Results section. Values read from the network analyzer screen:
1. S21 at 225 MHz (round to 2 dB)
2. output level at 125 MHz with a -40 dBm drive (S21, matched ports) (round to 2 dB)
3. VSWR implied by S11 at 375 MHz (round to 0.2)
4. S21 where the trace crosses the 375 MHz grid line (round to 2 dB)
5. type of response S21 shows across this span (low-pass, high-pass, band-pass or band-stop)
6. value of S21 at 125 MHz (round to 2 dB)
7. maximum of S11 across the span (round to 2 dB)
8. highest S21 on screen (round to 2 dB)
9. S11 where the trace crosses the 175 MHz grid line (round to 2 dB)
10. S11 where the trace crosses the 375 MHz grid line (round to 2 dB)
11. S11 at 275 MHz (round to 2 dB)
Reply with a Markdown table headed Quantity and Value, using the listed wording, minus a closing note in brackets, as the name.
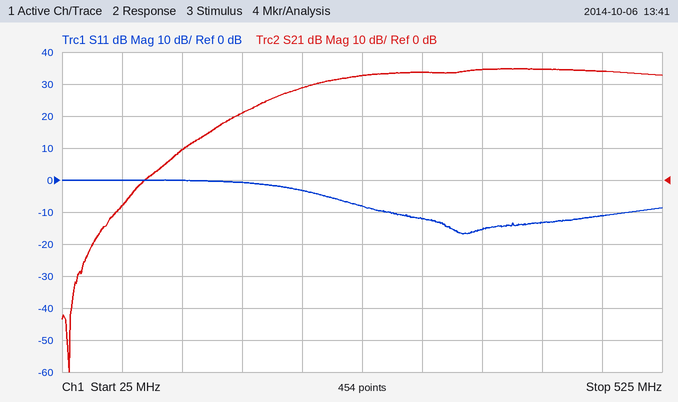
| Quantity | Value |
|---|---|
| S21 at 225 MHz | 28 dB |
| output level at 125 MHz with a -40 dBm drive (S21, matched ports) | -30 dBm |
| VSWR implied by S11 at 375 MHz | 1.4 |
| S21 where the trace crosses the 375 MHz grid line | 34 dB |
| type of response S21 shows across this span | high-pass |
| value of S21 at 125 MHz | 10 dB |
| maximum of S11 across the span | 0 dB |
| highest S21 on screen | 34 dB |
| S11 where the trace crosses the 175 MHz grid line | 0 dB |
| S11 where the trace crosses the 375 MHz grid line | -16 dB |
| S11 at 275 MHz | -8 dB |
